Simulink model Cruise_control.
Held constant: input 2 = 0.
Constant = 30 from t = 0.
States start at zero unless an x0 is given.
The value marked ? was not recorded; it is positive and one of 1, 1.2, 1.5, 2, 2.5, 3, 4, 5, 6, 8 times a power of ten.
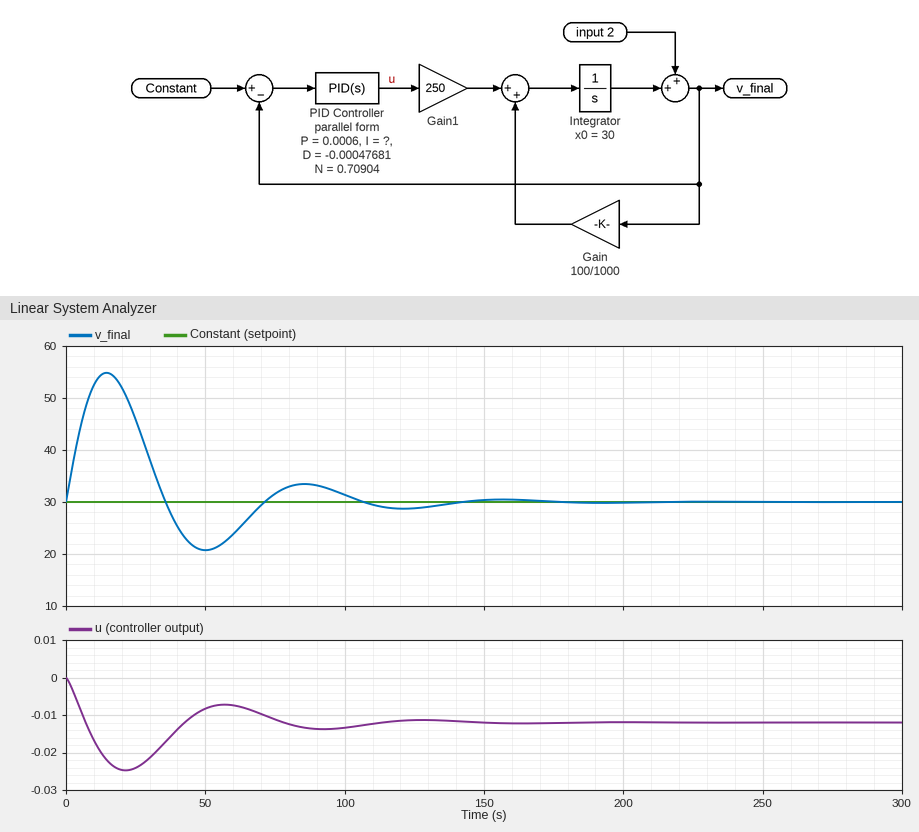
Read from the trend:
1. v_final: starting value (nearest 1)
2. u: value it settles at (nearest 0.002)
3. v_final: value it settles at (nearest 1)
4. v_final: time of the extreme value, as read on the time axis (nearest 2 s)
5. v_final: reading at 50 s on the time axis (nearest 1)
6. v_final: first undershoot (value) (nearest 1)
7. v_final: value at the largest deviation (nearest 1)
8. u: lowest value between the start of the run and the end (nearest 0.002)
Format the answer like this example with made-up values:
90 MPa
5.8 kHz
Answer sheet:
30
-0.012
30
14 s
21
21
55
-0.024
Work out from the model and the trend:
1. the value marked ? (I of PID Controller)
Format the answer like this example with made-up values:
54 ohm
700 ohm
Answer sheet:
3e-05
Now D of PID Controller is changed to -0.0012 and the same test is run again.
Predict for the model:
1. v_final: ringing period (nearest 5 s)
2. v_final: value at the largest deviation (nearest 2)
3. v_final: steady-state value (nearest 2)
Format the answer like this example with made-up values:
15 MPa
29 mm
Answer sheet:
65 s
58
30
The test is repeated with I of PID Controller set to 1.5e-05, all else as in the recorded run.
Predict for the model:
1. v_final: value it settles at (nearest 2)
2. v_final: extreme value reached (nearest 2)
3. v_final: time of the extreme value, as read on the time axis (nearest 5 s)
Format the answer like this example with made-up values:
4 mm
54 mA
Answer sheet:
30
60
20 s
